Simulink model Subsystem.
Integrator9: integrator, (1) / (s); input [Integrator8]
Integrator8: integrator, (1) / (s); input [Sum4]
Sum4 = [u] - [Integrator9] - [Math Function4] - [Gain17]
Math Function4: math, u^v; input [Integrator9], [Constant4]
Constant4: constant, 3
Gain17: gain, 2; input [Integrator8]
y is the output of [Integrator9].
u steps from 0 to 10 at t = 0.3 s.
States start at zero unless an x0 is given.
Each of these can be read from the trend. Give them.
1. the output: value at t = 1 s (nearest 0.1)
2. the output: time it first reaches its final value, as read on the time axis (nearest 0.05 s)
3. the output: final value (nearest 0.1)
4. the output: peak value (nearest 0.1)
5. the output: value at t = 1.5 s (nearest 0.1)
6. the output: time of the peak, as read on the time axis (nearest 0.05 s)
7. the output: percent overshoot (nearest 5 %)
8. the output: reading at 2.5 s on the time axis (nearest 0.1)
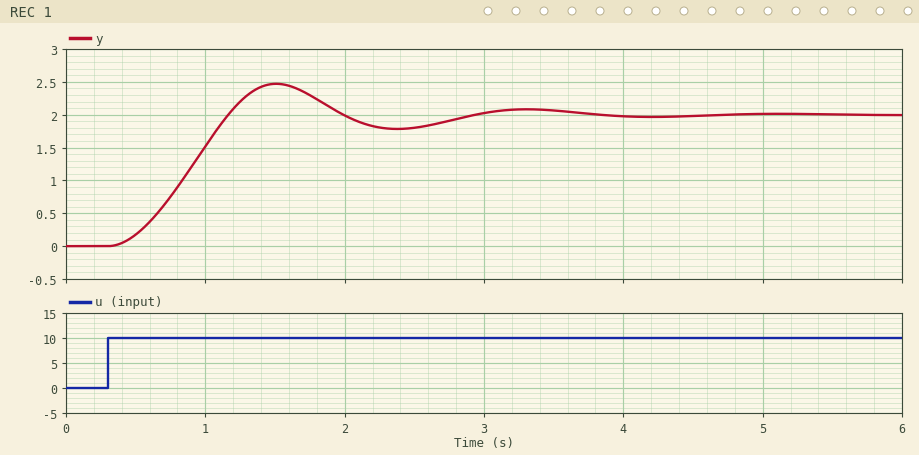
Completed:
1.5
1.15 s
2.0
2.5
2.5
1.50 s
25 %
1.8
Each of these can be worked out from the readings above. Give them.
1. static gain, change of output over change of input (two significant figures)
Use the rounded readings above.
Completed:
0.20
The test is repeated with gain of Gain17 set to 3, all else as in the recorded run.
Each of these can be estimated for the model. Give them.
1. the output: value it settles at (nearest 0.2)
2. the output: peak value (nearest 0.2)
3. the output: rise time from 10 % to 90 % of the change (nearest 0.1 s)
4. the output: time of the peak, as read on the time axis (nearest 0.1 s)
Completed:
2.0
2.2
0.7 s
1.7 s
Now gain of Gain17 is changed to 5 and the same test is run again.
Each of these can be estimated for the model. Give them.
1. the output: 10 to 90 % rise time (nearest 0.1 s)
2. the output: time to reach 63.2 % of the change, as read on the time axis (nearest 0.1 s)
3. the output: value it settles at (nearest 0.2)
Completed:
1.1 s
1.2 s
2.0
